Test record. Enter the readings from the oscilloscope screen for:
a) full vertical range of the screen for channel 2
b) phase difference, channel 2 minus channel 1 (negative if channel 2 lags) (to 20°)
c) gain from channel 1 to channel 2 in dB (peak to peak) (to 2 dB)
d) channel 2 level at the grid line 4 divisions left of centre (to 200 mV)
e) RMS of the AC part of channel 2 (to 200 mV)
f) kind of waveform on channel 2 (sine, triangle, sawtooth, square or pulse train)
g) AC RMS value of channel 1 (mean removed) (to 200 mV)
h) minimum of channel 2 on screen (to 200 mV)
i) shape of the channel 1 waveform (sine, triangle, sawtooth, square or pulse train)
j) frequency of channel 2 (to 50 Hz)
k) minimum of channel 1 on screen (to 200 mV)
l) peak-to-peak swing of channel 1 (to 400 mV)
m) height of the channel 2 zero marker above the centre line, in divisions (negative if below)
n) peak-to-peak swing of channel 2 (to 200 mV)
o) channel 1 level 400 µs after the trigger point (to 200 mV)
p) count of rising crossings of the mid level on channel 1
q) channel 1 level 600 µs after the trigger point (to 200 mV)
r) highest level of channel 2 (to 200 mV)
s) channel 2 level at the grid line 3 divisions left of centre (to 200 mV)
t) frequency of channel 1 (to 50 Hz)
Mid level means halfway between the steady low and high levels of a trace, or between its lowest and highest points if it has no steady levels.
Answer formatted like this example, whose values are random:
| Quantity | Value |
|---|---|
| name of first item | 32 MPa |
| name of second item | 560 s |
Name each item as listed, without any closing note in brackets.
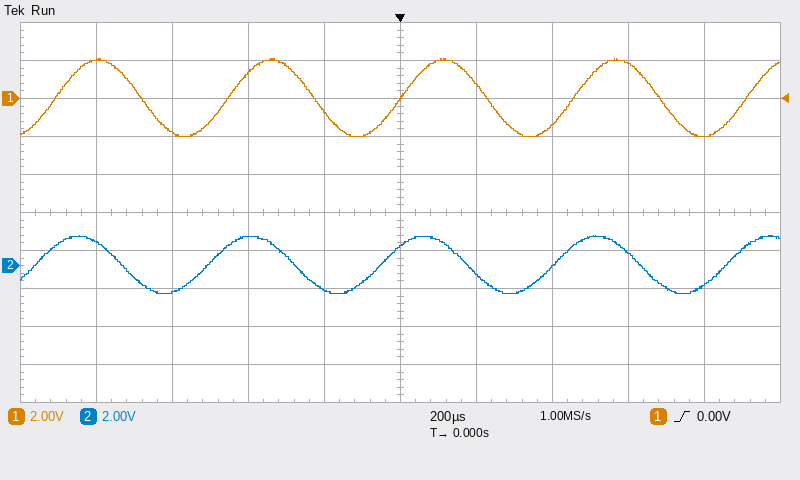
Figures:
| Quantity | Value |
|---|---|
| full vertical range of the screen for channel 2 | 20 V |
| phase difference, channel 2 minus channel 1 (negative if channel 2 lags) | +40° |
| gain from channel 1 to channel 2 in dB (peak to peak) | -2 dB |
| channel 2 level at the grid line 4 divisions left of centre | 1.2 V |
| RMS of the AC part of channel 2 | 1.0 V |
| kind of waveform on channel 2 | sine |
| AC RMS value of channel 1 (mean removed) | 1.4 V |
| minimum of channel 2 on screen | -1.4 V |
| shape of the channel 1 waveform | sine |
| frequency of channel 2 | 2.20 kHz |
| minimum of channel 1 on screen | -2.0 V |
| peak-to-peak swing of channel 1 | 4.0 V |
| height of the channel 2 zero marker above the centre line, in divisions | -1.4 div |
| peak-to-peak swing of channel 2 | 3.0 V |
| channel 1 level 400 µs after the trigger point | -1.4 V |
| count of rising crossings of the mid level on channel 1 | 5 |
| channel 1 level 600 µs after the trigger point | 1.8 V |
| highest level of channel 2 | 1.6 V |
| channel 2 level at the grid line 3 divisions left of centre | -1.4 V |
| frequency of channel 1 | 2.20 kHz |
